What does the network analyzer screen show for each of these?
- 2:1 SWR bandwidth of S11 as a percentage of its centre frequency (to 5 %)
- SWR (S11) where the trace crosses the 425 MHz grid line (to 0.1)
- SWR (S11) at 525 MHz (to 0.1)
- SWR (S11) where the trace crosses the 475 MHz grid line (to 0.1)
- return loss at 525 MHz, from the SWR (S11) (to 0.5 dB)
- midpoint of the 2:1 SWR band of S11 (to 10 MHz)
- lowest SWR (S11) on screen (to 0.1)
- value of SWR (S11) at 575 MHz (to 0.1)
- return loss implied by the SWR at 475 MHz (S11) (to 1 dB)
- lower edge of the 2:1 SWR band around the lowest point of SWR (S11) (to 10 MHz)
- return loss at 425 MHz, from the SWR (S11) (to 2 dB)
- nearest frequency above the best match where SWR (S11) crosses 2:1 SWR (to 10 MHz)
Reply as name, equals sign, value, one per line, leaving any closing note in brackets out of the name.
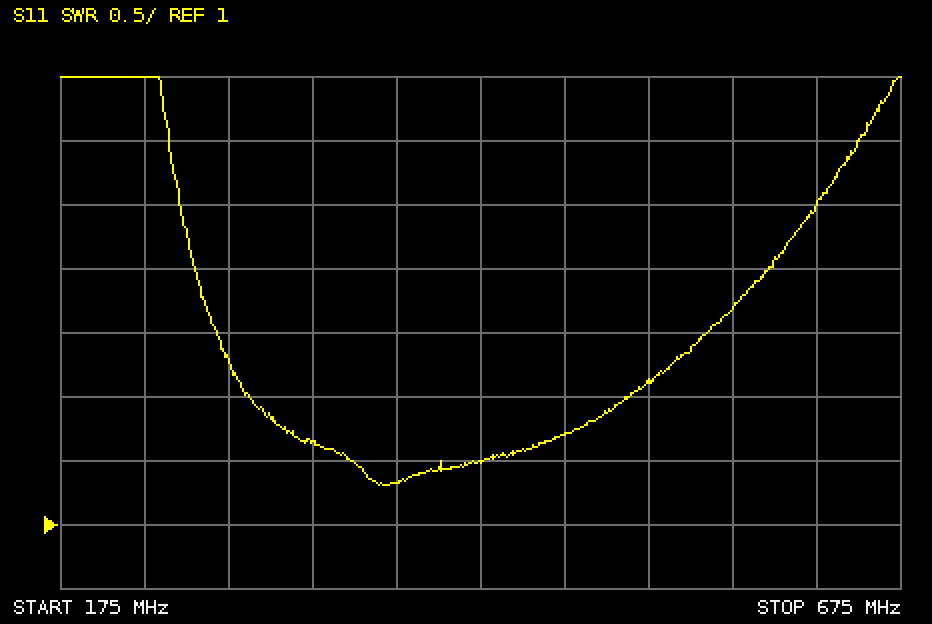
2:1 SWR bandwidth of S11 as a percentage of its centre frequency = 55 %
SWR (S11) where the trace crosses the 425 MHz grid line = 1.5
SWR (S11) at 525 MHz = 2.1
SWR (S11) where the trace crosses the 475 MHz grid line = 1.7
return loss at 525 MHz, from the SWR (S11) = 9.0 dB
midpoint of the 2:1 SWR band of S11 = 400 MHz
lowest SWR (S11) on screen = 1.3
value of SWR (S11) at 575 MHz = 2.7
return loss implied by the SWR at 475 MHz (S11) = 12 dB
lower edge of the 2:1 SWR band around the lowest point of SWR (S11) = 290 MHz
return loss at 425 MHz, from the SWR (S11) = 14 dB
nearest frequency above the best match where SWR (S11) crosses 2:1 SWR = 510 MHz
